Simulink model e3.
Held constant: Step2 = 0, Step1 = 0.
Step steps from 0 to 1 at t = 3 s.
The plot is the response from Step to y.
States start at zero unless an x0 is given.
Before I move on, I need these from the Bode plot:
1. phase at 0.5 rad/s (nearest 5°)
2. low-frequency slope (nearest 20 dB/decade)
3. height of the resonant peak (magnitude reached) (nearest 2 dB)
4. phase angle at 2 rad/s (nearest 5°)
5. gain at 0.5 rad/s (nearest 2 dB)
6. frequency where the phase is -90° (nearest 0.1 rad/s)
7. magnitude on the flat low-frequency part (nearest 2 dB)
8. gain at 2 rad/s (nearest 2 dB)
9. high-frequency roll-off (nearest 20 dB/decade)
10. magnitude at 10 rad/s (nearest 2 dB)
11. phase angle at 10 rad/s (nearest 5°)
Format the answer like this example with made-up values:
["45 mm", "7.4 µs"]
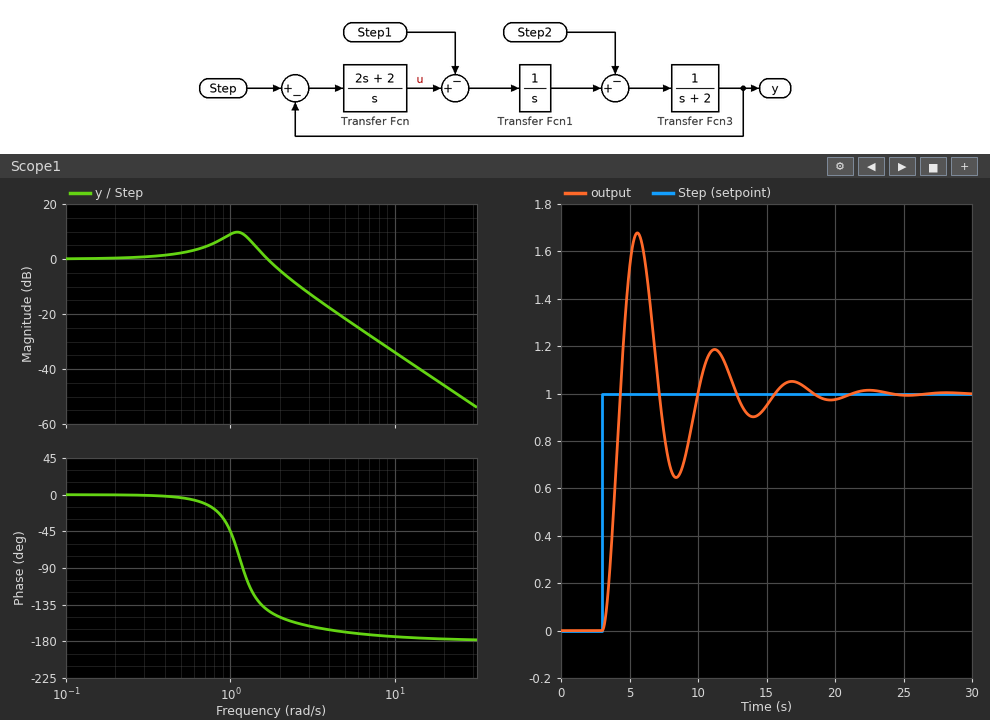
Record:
["-5°", "0 dB/decade", "10 dB", "-150°", "2 dB", "1.2 rad/s", "0 dB", "-4 dB", "-40 dB/decade", "-34 dB", "-175°"]
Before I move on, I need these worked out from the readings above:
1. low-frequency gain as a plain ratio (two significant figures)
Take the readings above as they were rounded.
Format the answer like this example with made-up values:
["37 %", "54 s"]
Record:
["1.0"]
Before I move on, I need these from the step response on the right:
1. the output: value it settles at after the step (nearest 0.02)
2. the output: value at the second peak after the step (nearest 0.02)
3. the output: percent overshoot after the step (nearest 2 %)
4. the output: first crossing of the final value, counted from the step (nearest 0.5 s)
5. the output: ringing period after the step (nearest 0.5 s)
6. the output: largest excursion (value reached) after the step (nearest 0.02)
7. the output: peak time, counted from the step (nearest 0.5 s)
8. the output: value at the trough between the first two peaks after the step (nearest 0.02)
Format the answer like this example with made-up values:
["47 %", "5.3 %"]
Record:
["1.00", "1.18", "68 %", "1.5 s", "5.5 s", "1.68", "2.5 s", "0.64"]
